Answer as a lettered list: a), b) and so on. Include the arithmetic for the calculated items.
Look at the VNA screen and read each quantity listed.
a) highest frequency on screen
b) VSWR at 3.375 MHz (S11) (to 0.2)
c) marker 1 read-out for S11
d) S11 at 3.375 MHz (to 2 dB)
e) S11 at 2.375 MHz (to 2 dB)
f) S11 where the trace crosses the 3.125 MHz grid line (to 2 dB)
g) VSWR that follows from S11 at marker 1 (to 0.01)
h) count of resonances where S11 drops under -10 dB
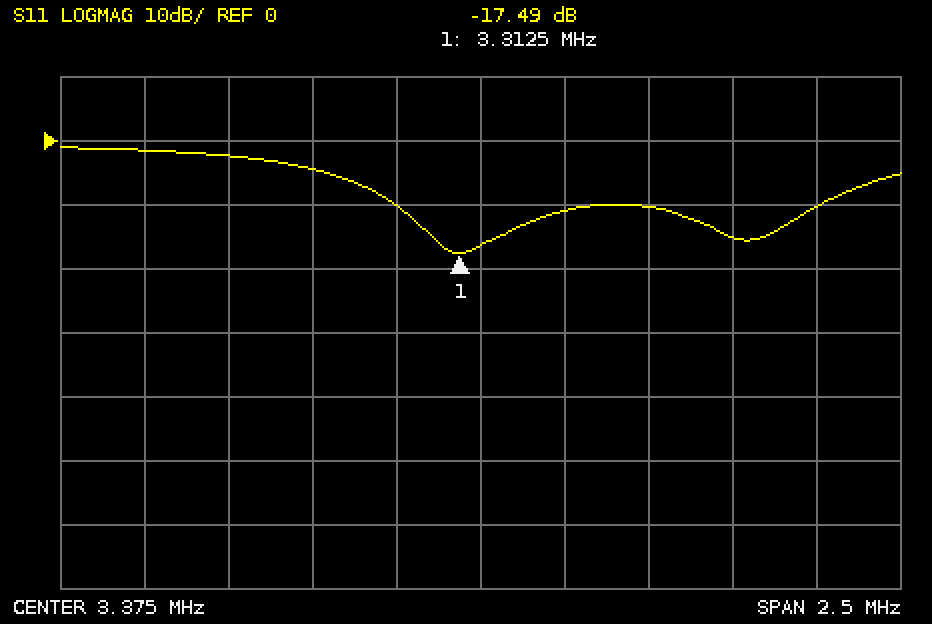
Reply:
a) 4.625 MHz
b) |Γ| = 10^(-16/20) = 0.1585; VSWR = (1 + 0.1585)/(1 − 0.1585) ≈ 1.4
c) -17.49 dB
d) -16 dB
e) -2 dB
f) -10 dB
g) (1 + 0.1335)/(1 − 0.1335) ≈ 1.31
h) 2
